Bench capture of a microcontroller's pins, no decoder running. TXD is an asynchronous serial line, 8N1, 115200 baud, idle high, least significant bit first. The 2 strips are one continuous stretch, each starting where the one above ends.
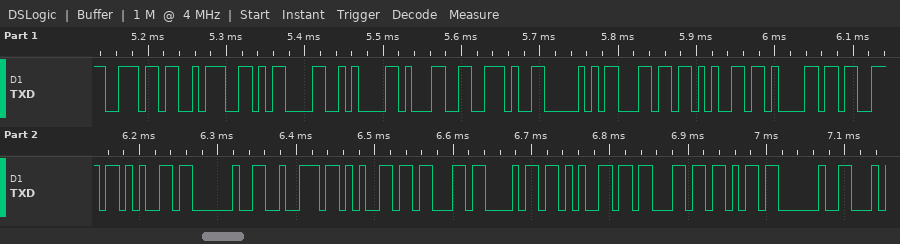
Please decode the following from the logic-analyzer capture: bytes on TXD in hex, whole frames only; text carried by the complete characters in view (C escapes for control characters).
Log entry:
6E 3A 0D 0A 31 2E 50 6C 65 61 73 65 20 72 65 63 68 65 63 6B 20
"n:\r\n1.Please recheck "
